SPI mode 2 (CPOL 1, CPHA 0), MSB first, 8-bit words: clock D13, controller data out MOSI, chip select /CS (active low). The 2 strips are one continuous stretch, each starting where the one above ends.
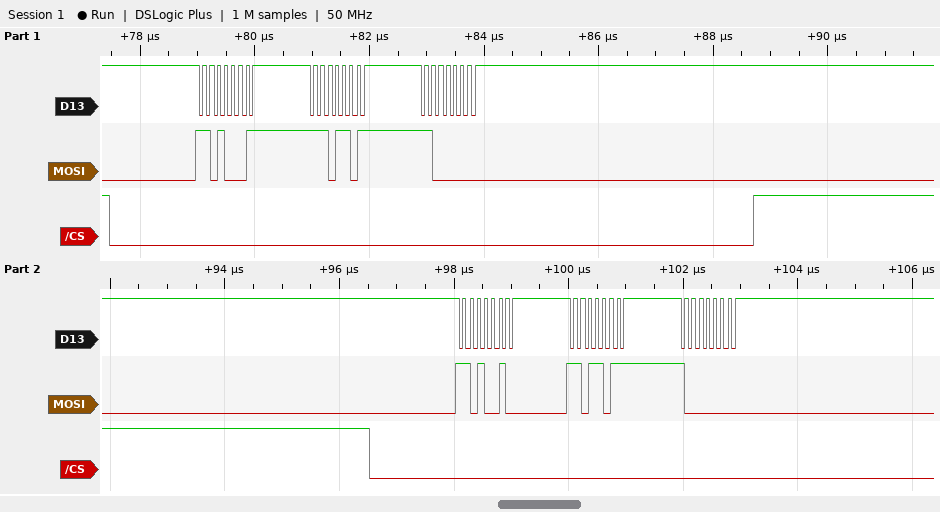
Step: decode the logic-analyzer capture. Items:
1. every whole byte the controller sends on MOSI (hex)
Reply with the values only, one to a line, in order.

D1 ED C0 D2 DB 80
